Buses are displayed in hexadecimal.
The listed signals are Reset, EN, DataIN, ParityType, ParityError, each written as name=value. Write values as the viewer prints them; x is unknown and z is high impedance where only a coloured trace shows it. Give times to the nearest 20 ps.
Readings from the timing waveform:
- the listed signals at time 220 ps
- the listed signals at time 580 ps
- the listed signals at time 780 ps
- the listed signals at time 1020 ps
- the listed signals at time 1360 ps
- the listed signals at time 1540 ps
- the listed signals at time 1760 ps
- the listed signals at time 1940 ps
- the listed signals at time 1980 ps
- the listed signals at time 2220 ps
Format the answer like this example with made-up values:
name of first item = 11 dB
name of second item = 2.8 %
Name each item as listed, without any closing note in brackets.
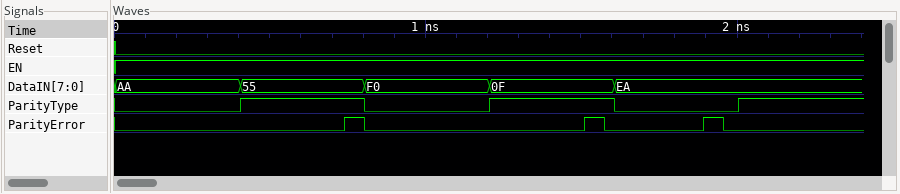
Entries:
the listed signals at time 220 ps = Reset=0, EN=1, DataIN=AA, ParityType=0, ParityError=0
the listed signals at time 580 ps = Reset=0, EN=1, DataIN=55, ParityType=1, ParityError=0
the listed signals at time 780 ps = Reset=0, EN=1, DataIN=55, ParityType=1, ParityError=1
the listed signals at time 1020 ps = Reset=0, EN=1, DataIN=F0, ParityType=0, ParityError=0
the listed signals at time 1360 ps = Reset=0, EN=1, DataIN=0F, ParityType=1, ParityError=0
the listed signals at time 1540 ps = Reset=0, EN=1, DataIN=0F, ParityType=1, ParityError=1
the listed signals at time 1760 ps = Reset=0, EN=1, DataIN=EA, ParityType=0, ParityError=0
the listed signals at time 1940 ps = Reset=0, EN=1, DataIN=EA, ParityType=0, ParityError=1
the listed signals at time 1980 ps = Reset=0, EN=1, DataIN=EA, ParityType=0, ParityError=0
the listed signals at time 2220 ps = Reset=0, EN=1, DataIN=EA, ParityType=1, ParityError=0
